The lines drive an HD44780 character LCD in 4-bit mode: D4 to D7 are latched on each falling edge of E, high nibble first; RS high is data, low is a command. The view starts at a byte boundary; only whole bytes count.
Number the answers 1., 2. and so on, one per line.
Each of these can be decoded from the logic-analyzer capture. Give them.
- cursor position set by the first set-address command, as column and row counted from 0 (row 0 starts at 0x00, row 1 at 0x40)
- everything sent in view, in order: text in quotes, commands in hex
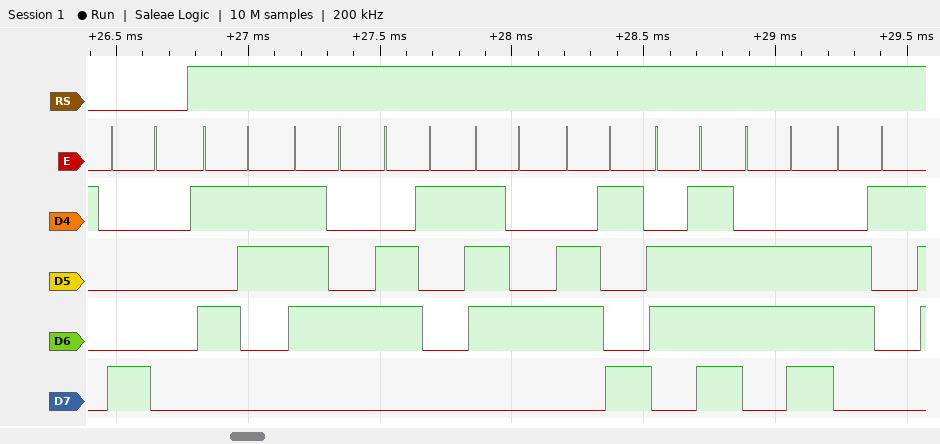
1. column 0, row 0
2. 0x80 "Stationa"
